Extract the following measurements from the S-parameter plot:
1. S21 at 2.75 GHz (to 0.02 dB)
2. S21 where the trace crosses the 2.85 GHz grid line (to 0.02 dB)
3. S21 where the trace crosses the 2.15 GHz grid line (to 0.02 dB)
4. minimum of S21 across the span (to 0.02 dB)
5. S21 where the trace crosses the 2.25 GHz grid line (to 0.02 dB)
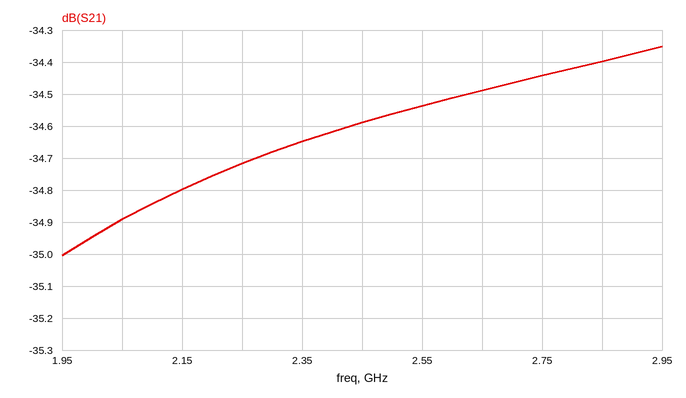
-34.44 dB
-34.40 dB
-34.80 dB
-35.00 dB
-34.72 dB
